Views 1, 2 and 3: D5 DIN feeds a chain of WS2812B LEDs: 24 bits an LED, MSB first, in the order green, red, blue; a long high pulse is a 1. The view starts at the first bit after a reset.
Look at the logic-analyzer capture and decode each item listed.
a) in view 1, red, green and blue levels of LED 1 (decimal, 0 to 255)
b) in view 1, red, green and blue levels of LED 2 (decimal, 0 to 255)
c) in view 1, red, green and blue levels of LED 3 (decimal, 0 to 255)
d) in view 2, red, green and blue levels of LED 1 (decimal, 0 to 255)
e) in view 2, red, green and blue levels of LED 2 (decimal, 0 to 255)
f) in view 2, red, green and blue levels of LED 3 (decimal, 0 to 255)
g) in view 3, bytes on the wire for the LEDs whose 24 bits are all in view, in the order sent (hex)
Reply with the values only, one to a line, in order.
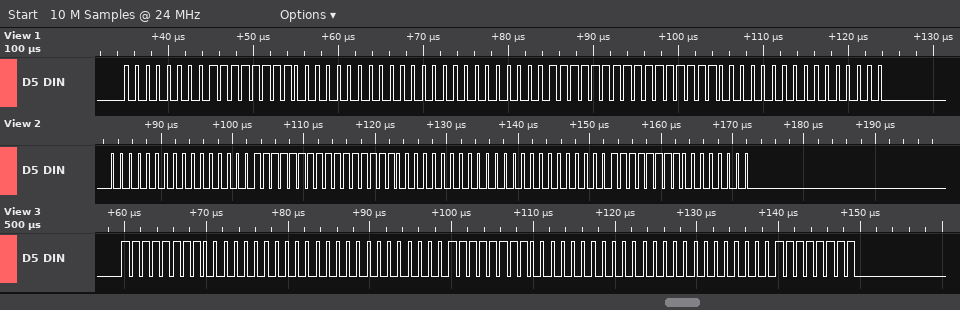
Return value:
255, 0, 0
0, 0, 255
0, 255, 0
0, 0, 255
0, 255, 0
255, 0, 0
FF 00 00 00 FF 00 00 00 FF
